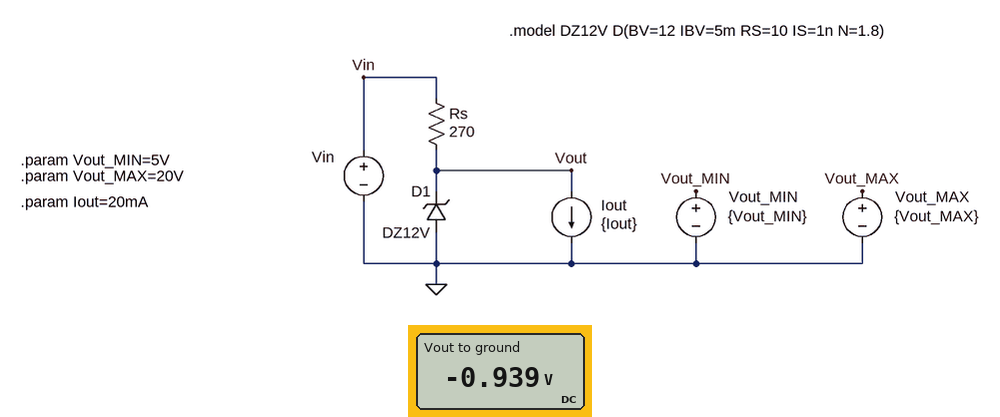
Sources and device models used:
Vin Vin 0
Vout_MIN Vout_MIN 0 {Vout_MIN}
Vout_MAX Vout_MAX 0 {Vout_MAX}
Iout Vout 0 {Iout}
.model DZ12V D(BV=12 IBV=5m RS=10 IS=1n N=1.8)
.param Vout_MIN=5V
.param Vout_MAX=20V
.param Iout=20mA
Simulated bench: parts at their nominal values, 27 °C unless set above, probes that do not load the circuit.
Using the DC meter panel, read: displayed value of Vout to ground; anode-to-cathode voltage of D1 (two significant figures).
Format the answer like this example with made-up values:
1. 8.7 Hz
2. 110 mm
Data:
1. -0.939 V
2. 940 mV
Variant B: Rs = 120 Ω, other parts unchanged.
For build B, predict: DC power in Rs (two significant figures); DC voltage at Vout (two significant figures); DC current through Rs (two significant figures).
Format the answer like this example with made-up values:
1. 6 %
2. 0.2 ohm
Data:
1. 6.6 mW
2. -890 mV
3. 7.4 mA
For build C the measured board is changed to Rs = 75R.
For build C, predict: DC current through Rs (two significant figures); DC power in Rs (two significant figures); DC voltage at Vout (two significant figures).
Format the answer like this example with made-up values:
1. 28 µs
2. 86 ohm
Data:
1. 11 mA
2. 9.3 mW
3. -830 mV
